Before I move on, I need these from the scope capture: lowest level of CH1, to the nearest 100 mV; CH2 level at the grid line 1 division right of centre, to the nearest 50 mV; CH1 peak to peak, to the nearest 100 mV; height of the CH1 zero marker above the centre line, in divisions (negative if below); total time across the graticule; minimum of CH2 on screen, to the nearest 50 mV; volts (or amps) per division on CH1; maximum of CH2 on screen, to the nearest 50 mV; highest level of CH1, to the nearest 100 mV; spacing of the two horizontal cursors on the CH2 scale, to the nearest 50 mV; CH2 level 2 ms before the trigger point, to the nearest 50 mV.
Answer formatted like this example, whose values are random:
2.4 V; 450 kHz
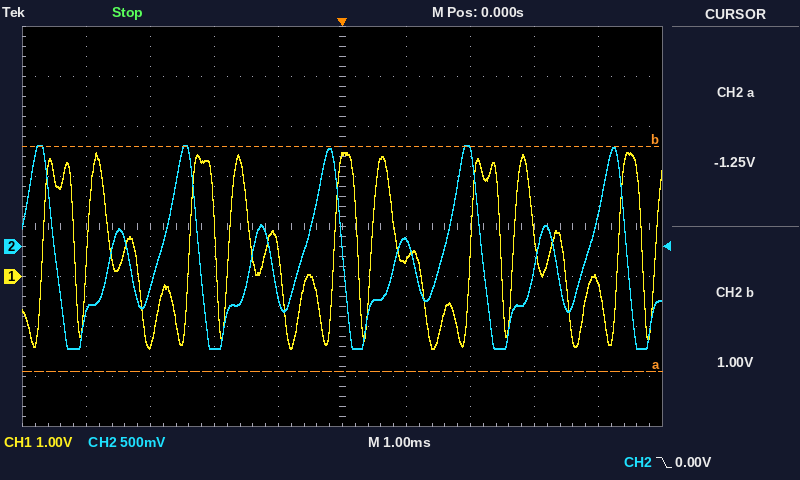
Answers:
-1.4 V; 50 mV; 3.9 V; -1.0 div; 10 ms; -1.00 V; 1 V; 1.00 V; 2.5 V; 2.25 V; -1.00 V
